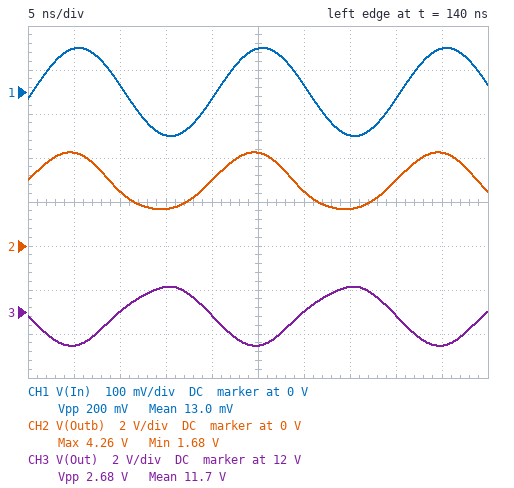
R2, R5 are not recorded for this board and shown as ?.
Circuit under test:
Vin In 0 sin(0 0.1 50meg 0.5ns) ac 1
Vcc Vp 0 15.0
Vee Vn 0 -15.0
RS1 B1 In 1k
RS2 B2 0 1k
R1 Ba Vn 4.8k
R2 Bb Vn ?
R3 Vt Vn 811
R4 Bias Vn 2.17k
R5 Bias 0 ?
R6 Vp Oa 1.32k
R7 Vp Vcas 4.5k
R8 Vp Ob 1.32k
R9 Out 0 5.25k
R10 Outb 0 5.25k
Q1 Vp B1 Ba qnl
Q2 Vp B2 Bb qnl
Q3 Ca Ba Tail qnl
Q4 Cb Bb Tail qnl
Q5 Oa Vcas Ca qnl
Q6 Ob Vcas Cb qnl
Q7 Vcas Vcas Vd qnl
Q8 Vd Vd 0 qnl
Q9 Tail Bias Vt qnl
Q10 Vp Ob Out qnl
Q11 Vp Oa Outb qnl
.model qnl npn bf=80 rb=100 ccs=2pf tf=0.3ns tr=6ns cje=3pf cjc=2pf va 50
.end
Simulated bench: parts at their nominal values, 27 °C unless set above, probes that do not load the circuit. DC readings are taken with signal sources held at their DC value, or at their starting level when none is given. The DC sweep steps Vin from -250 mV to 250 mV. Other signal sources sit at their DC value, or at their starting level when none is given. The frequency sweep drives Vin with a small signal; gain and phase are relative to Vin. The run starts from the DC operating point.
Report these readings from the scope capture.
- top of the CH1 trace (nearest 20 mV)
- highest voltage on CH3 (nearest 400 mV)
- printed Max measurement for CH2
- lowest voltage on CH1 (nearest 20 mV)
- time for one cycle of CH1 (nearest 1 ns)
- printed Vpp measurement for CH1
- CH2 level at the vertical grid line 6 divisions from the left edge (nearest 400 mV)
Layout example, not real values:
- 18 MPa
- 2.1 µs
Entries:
- 100 mV
- 13.2 V
- 4.26 V
- -100 mV
- 20 ns
- 200 mV
- 2.4 V
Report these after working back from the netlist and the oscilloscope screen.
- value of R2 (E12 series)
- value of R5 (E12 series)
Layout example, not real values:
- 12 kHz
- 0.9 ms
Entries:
- 1.8 kΩ
- 1.2 kΩ
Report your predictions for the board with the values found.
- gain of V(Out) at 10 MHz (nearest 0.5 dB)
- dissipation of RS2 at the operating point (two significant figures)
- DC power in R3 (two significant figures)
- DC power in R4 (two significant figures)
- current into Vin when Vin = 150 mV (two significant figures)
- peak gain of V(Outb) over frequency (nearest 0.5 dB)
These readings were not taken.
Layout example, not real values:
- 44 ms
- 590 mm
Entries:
- 30.5 dB
- 5.6 µW
- 94 mW
- 42 mW
- -30 µA
- 31.0 dB
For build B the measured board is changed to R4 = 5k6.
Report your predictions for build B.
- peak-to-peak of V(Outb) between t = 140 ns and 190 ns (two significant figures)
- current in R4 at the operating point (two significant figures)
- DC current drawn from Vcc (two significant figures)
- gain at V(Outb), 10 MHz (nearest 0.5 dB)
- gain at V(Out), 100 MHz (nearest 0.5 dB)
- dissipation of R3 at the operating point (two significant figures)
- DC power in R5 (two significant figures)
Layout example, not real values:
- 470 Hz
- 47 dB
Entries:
- 450 mV
- 2.2 mA
- 28 mA
- 11.5 dB
- 6.5 dB
- 160 mW
- 6.6 mW
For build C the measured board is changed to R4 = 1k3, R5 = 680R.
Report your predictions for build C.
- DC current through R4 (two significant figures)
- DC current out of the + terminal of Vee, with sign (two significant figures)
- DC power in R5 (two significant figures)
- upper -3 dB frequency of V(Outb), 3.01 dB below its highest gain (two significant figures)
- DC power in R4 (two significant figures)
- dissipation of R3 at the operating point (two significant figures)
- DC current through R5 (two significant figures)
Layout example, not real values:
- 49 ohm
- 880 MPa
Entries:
- 7.5 mA
- -29 mA
- 40 mW
- 29 MHz
- 74 mW
- 99 mW
- 7.7 mA
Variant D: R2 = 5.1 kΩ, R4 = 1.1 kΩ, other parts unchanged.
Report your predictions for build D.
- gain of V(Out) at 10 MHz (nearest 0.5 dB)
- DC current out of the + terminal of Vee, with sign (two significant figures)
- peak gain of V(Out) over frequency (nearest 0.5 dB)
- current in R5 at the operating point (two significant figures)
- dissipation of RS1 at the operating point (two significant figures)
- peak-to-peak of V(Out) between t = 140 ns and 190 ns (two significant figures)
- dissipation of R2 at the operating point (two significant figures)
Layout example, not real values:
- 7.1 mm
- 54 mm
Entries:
- 37.5 dB
- -20 mA
- 38.0 dB
- 6.6 mA
- 810 nW
- 3.2 V
- 39 mW
